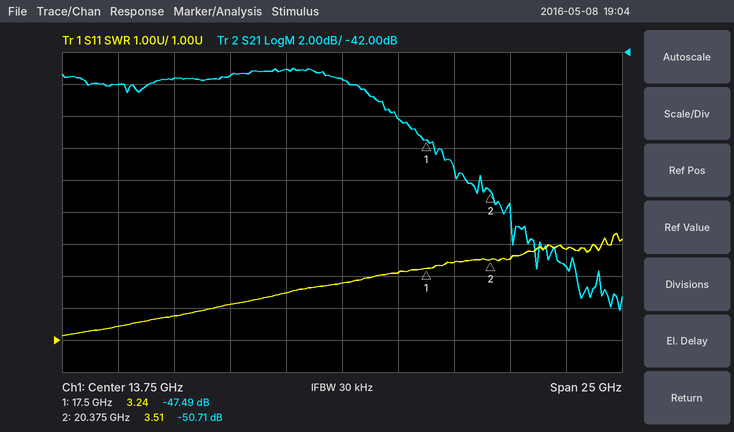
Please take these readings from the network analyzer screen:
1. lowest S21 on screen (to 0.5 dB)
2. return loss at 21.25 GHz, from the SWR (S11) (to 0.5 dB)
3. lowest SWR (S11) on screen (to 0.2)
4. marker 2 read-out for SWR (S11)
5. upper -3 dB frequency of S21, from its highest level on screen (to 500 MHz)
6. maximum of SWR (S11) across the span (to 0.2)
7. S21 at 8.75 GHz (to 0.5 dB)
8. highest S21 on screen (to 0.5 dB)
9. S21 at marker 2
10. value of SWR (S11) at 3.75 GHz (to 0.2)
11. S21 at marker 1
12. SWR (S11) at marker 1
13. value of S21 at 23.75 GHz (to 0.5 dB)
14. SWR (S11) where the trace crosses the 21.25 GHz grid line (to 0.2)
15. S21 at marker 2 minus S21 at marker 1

-58.0 dB
5.0 dB
1.2
3.51
16.0 GHz
4.4
-43.5 dB
-43.0 dB
-50.71 dB
1.4
-47.49 dB
3.24
-55.5 dB
3.6
-3.22 dB
